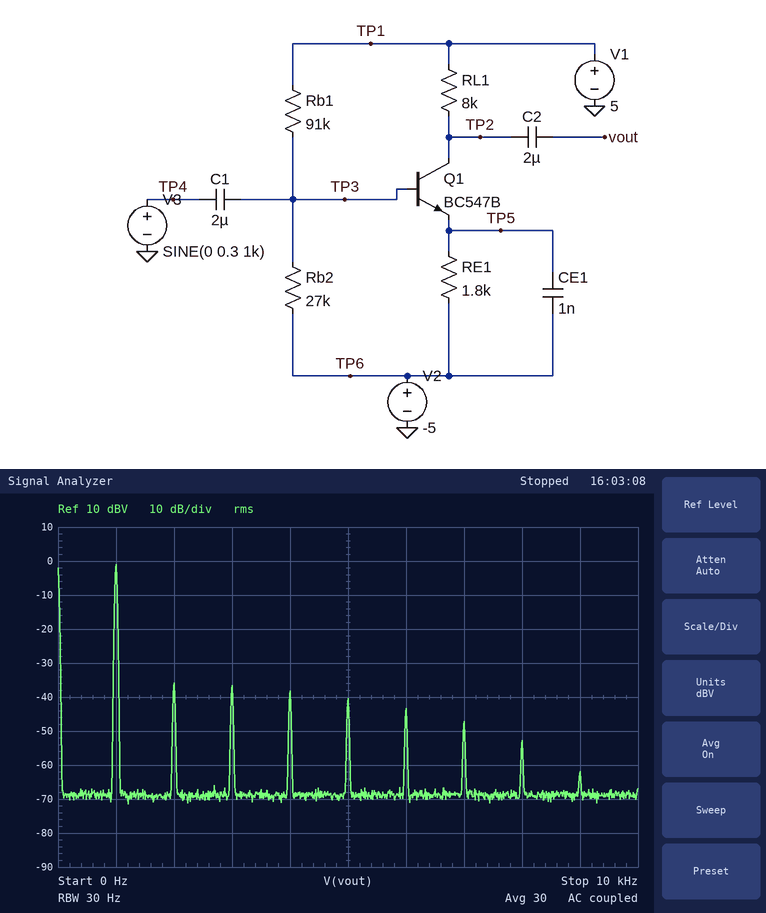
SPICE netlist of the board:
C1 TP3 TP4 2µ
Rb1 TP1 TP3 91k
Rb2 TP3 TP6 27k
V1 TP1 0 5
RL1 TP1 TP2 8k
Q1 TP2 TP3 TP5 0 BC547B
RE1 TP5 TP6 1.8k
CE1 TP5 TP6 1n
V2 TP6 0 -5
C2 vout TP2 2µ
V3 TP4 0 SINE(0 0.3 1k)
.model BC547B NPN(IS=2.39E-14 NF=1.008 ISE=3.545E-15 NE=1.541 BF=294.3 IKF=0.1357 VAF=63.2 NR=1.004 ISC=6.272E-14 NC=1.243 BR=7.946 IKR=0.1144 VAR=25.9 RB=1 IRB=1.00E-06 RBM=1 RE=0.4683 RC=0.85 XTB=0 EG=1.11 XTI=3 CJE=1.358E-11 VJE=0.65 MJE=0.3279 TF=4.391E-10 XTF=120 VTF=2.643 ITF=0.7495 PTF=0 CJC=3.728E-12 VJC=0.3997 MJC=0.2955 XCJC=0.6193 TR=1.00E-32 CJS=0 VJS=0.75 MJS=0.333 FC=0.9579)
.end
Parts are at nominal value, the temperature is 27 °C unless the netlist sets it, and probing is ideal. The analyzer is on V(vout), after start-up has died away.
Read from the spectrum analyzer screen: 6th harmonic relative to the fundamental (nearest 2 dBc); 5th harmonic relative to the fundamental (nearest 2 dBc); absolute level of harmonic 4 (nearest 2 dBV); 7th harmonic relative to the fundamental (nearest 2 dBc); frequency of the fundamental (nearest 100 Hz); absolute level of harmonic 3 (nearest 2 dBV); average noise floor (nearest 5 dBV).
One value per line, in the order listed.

-42 dBc
-40 dBc
-38 dBV
-46 dBc
1.0 kHz
-36 dBV
-70 dBV
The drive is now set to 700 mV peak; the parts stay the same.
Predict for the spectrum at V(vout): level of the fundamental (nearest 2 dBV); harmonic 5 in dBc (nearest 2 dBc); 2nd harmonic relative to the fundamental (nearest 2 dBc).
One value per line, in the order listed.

6 dBV
-34 dBc
-24 dBc
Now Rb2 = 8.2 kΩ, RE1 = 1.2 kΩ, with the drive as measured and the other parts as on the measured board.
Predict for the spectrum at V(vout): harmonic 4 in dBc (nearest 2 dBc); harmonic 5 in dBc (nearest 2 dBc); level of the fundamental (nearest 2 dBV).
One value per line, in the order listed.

-42 dBc
-50 dBc
2 dBV
